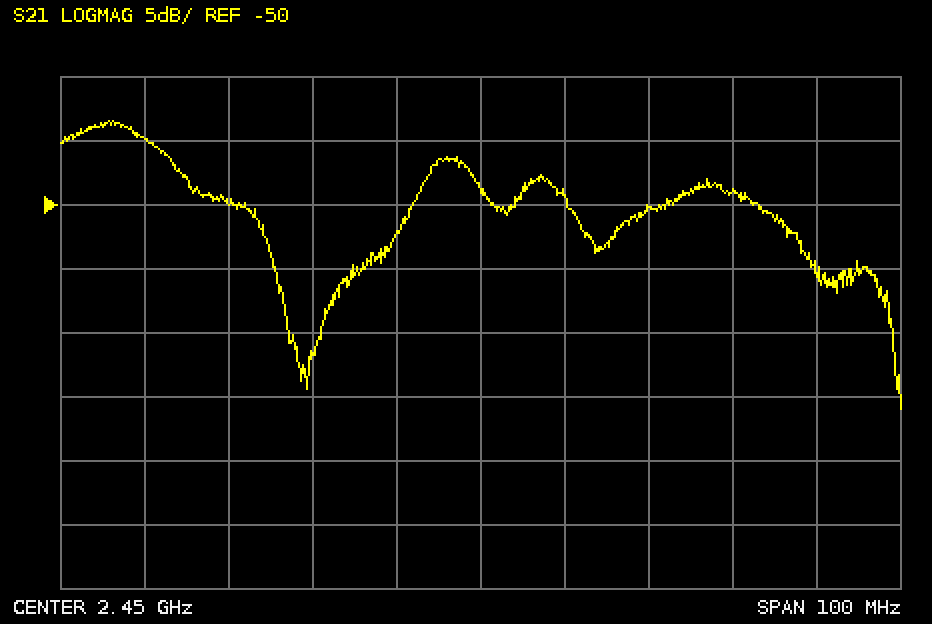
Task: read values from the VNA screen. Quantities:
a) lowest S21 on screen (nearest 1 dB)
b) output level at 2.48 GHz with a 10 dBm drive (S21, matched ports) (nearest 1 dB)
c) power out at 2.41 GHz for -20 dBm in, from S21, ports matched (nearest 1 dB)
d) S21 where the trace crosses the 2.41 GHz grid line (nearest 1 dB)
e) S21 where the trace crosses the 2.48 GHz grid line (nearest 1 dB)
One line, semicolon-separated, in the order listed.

-66 dB; -39 dBm; -65 dBm; -45 dB; -49 dB
